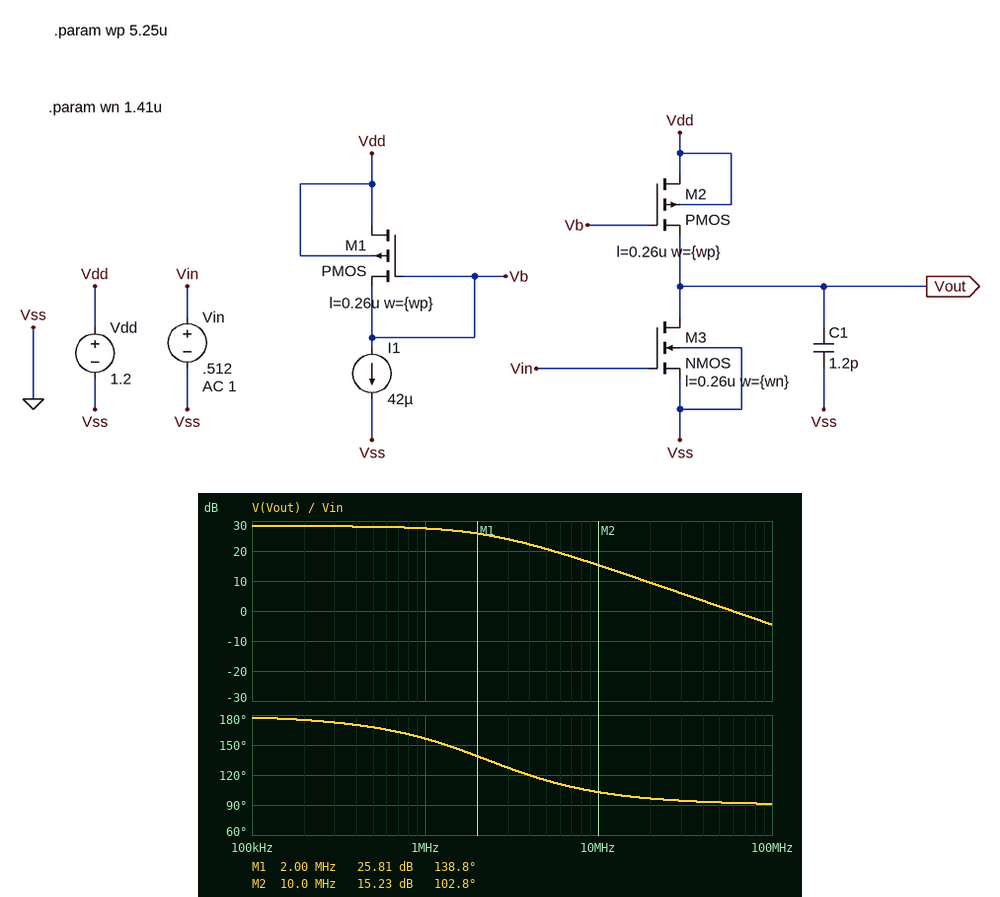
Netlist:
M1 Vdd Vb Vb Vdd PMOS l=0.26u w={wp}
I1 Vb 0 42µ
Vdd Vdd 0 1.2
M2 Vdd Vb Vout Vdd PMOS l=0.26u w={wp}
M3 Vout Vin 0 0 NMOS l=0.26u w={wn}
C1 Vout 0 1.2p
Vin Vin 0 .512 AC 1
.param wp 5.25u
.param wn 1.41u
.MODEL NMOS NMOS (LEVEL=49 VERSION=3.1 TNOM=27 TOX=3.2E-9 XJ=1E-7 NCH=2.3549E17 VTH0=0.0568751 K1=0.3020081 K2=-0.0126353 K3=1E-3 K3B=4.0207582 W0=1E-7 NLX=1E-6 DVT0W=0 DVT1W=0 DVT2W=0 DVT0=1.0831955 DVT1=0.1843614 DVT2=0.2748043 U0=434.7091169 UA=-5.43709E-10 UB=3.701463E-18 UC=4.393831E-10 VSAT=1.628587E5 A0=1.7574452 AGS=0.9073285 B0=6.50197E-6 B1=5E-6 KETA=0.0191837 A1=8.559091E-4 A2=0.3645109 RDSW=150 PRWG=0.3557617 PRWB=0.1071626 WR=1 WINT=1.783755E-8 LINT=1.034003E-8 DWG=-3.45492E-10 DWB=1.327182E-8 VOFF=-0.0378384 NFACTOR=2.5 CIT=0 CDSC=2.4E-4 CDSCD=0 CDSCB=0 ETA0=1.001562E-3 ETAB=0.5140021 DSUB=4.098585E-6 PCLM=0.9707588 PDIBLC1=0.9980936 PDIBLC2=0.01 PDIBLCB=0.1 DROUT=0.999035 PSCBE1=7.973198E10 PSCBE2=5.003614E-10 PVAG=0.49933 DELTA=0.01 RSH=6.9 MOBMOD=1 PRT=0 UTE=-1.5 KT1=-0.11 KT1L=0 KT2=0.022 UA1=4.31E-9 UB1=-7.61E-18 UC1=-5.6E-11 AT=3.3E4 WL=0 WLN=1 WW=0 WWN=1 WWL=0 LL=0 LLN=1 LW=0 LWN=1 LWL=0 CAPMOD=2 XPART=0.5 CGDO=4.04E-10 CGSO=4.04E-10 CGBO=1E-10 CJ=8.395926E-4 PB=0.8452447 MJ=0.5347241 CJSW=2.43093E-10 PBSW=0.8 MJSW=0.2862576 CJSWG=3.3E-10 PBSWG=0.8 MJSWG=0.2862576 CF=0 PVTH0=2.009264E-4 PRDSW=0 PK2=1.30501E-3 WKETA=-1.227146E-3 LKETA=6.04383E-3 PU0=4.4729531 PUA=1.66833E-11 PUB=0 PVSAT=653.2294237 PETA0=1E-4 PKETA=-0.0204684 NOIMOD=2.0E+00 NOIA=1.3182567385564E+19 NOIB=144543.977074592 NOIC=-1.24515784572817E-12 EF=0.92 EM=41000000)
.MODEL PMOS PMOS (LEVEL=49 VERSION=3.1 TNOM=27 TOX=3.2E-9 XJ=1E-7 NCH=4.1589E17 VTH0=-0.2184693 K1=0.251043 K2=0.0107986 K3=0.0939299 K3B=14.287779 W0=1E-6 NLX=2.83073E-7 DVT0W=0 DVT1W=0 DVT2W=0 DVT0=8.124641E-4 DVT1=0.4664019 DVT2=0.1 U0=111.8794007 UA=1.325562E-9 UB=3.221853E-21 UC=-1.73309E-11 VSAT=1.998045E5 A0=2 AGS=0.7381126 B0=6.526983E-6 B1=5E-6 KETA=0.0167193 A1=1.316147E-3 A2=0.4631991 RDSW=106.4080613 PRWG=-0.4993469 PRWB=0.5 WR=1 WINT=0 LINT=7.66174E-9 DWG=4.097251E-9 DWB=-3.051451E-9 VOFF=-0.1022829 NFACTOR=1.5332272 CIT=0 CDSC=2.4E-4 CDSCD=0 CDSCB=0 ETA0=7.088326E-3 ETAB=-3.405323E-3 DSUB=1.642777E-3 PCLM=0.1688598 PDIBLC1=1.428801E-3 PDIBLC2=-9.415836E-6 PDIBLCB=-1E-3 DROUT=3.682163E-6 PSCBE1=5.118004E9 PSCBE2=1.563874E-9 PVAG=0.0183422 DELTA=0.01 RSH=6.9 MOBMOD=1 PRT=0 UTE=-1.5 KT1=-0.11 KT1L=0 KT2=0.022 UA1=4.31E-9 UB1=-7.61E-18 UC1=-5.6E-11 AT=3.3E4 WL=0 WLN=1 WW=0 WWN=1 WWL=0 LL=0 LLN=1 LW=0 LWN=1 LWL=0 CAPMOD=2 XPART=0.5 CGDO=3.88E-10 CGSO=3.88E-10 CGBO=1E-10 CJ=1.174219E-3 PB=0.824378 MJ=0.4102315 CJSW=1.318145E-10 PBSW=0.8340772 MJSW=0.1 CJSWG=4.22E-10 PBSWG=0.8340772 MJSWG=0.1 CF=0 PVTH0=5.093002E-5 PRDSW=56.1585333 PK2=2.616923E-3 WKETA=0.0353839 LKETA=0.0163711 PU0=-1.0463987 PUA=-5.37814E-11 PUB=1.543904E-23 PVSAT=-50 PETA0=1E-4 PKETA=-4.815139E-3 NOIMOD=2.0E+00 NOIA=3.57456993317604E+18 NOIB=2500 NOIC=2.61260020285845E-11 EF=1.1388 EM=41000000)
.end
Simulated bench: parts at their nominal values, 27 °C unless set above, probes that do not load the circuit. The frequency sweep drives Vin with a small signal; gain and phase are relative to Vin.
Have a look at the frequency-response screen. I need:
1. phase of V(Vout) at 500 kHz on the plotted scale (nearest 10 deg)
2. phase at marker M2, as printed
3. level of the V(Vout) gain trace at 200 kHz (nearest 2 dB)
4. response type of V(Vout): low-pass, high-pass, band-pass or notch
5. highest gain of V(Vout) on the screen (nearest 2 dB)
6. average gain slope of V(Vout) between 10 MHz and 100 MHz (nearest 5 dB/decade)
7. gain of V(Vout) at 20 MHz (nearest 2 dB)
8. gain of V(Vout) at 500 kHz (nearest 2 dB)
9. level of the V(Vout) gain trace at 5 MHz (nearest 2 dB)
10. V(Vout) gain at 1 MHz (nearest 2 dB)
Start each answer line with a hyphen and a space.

- 170 deg
- 102.8 deg
- 28 dB
- low-pass
- 28 dB
- -20 dB/decade
- 10 dB
- 28 dB
- 20 dB
- 28 dB
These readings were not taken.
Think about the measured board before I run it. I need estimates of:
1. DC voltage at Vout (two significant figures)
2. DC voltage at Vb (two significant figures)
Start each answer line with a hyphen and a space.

- 620 mV
- 670 mV
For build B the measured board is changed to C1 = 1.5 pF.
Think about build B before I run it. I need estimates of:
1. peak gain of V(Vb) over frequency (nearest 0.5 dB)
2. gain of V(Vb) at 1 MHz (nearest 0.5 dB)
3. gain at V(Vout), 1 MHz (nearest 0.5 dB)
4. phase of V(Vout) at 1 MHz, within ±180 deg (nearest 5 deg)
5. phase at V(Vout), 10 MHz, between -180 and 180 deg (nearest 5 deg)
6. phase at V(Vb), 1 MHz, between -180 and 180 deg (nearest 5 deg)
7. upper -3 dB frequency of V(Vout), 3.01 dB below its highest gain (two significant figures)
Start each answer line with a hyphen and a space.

- -56.5 dB
- -63.0 dB
- 27.0 dB
- 150 deg
- 100 deg
- -120 deg
- 1.8 MHz
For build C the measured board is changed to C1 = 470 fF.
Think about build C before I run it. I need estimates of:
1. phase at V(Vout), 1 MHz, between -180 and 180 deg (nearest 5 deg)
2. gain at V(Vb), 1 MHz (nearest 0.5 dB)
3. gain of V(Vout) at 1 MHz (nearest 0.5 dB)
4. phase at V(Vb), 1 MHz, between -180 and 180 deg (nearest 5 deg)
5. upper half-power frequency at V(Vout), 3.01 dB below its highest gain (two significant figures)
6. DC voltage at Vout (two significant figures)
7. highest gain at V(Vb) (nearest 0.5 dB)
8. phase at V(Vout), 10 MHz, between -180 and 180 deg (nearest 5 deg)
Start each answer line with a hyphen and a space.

- 170 deg
- -62.0 dB
- 28.0 dB
- -100 deg
- 5.8 MHz
- 620 mV
- -46.5 dB
- 120 deg
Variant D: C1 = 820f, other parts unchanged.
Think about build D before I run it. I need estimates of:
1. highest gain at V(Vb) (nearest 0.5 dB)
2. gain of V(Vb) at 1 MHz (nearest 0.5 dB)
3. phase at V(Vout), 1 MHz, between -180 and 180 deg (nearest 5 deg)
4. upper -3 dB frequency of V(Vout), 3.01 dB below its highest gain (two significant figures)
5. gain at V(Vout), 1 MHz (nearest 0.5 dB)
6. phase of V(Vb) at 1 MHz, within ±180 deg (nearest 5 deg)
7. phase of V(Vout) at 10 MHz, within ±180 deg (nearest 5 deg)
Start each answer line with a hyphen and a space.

- -51.5 dB
- -62.0 dB
- 165 deg
- 3.3 MHz
- 28.0 dB
- -105 deg
- 110 deg
